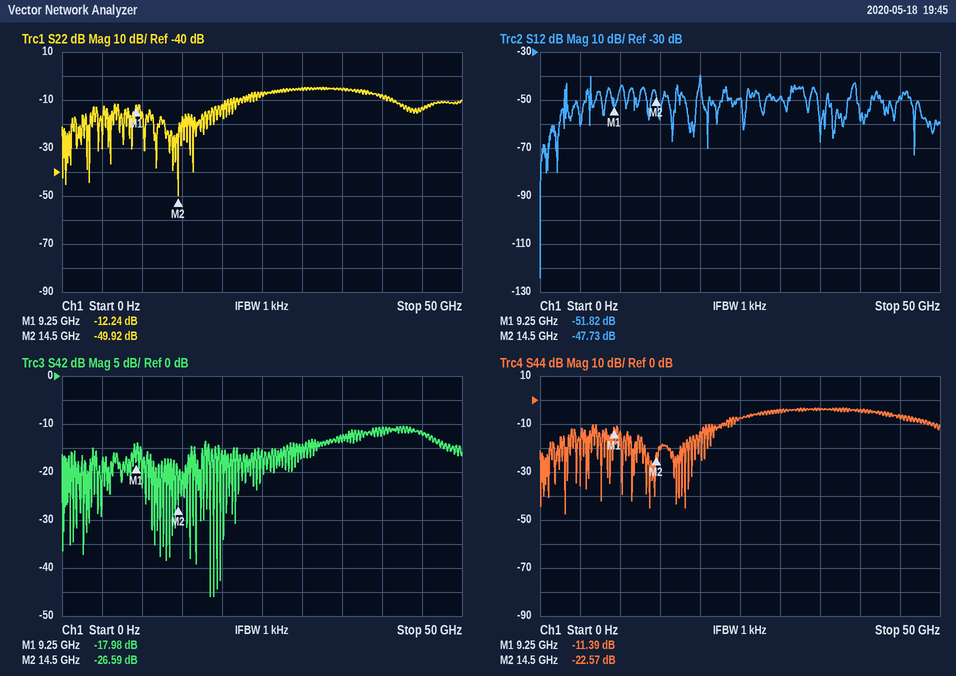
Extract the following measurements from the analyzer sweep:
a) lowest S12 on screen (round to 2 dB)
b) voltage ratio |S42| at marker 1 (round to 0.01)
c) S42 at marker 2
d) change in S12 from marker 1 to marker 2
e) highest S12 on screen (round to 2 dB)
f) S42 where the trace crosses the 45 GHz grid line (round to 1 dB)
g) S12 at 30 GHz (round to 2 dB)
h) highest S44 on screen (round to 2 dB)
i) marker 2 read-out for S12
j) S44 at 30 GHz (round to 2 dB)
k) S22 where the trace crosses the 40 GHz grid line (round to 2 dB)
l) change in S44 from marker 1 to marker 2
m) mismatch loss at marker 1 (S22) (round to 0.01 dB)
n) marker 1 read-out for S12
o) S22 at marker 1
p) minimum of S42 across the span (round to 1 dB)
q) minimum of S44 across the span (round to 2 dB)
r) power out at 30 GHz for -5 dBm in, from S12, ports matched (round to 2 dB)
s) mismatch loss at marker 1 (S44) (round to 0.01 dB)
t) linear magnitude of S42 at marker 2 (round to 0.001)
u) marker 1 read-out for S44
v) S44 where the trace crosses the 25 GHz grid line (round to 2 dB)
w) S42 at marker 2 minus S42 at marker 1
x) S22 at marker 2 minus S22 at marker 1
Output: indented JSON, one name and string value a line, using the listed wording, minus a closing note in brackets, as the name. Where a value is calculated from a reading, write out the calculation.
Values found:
{
  "lowest S12 on screen": "-124 dB",
  "voltage ratio |S42| at marker 1": "10^(-17.98/20) ≈ 0.13",
  "S42 at marker 2": "-26.59 dB",
  "change in S12 from marker 1 to marker 2": "-47.73 − (-51.82) = 4.09 dB",
  "highest S12 on screen": "-40 dB",
  "S42 where the trace crosses the 45 GHz grid line": "-12 dB",
  "S12 at 30 GHz": "-48 dB",
  "highest S44 on screen": "-4 dB",
  "marker 2 read-out for S12": "-47.73 dB",
  "S44 at 30 GHz": "-4 dB",
  "S22 where the trace crosses the 40 GHz grid line": "-8 dB",
  "change in S44 from marker 1 to marker 2": "-22.57 − (-11.39) = -11.18 dB",
  "mismatch loss at marker 1 (S22)": "−10 log10(1 − 10^(-12.24/10)) ≈ 0.27 dB",
  "marker 1 read-out for S12": "-51.82 dB",
  "S22 at marker 1": "-12.24 dB",
  "minimum of S42 across the span": "-46 dB",
  "minimum of S44 across the span": "-48 dB",
  "power out at 30 GHz for -5 dBm in, from S12, ports matched": "-5 dBm + (-48 dB) = -54 dBm",
  "mismatch loss at marker 1 (S44)": "−10 log10(1 − 10^(-11.39/10)) ≈ 0.33 dB",
  "linear magnitude of S42 at marker 2": "10^(-26.59/20) ≈ 0.047",
  "marker 1 read-out for S44": "-11.39 dB",
  "S44 where the trace crosses the 25 GHz grid line": "-8 dB",
  "S42 at marker 2 minus S42 at marker 1": "-26.59 − (-17.98) = -8.61 dB",
  "S22 at marker 2 minus S22 at marker 1": "-49.92 − (-12.24) = -37.68 dB"
}
